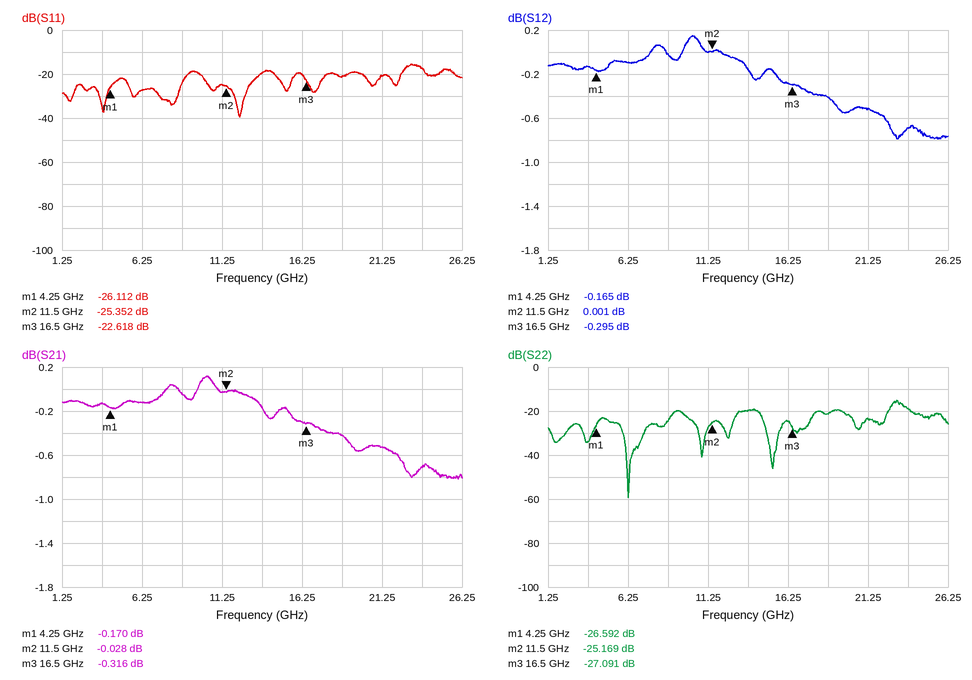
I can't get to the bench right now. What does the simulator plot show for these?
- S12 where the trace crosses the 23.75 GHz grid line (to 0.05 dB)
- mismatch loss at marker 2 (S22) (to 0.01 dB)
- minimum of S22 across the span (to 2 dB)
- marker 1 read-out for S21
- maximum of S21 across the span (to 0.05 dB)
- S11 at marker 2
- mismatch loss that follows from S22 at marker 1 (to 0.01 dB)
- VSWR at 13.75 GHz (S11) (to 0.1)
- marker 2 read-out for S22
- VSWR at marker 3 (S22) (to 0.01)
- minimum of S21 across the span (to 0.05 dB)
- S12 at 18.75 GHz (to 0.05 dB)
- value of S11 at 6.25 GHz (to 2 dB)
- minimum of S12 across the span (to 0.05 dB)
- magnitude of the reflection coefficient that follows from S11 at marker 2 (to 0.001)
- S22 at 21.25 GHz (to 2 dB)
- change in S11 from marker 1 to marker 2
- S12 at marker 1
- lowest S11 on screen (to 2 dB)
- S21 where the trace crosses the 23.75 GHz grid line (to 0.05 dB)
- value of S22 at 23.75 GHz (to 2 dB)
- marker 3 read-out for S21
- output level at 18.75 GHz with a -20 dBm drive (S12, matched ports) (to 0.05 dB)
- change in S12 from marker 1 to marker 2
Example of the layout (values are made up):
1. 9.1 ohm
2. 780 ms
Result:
1. -0.70 dB
2. 0.01 dB
3. -60 dB
4. -0.170 dB
5. 0.10 dB
6. -25.352 dB
7. 0.01 dB
8. 1.2
9. -25.169 dB
10. 1.09
11. -0.80 dB
12. -0.40 dB
13. -28 dB
14. -0.80 dB
15. 0.054
16. -24 dB
17. 0.760 dB
18. -0.165 dB
19. -40 dB
20. -0.70 dB
21. -18 dB
22. -0.316 dB
23. -20.40 dBm
24. 0.166 dB
